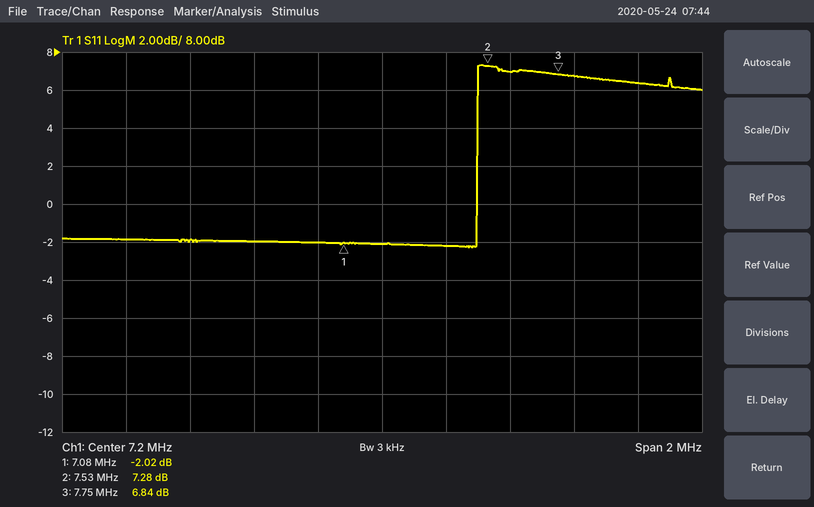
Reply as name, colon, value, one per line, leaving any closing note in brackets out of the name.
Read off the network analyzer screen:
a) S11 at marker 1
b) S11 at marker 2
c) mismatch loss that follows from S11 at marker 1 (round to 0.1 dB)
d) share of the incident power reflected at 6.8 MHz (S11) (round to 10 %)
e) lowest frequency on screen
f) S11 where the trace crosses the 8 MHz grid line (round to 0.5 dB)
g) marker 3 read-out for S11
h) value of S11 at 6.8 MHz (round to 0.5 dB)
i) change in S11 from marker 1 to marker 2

S11 at marker 1: -2.02 dB
S11 at marker 2: 7.28 dB
mismatch loss that follows from S11 at marker 1: 4.3 dB
share of the incident power reflected at 6.8 MHz (S11): 60 %
lowest frequency on screen: 6.2 MHz
S11 where the trace crosses the 8 MHz grid line: 6.5 dB
marker 3 read-out for S11: 6.84 dB
value of S11 at 6.8 MHz: -2.0 dB
change in S11 from marker 1 to marker 2: 9.30 dB
